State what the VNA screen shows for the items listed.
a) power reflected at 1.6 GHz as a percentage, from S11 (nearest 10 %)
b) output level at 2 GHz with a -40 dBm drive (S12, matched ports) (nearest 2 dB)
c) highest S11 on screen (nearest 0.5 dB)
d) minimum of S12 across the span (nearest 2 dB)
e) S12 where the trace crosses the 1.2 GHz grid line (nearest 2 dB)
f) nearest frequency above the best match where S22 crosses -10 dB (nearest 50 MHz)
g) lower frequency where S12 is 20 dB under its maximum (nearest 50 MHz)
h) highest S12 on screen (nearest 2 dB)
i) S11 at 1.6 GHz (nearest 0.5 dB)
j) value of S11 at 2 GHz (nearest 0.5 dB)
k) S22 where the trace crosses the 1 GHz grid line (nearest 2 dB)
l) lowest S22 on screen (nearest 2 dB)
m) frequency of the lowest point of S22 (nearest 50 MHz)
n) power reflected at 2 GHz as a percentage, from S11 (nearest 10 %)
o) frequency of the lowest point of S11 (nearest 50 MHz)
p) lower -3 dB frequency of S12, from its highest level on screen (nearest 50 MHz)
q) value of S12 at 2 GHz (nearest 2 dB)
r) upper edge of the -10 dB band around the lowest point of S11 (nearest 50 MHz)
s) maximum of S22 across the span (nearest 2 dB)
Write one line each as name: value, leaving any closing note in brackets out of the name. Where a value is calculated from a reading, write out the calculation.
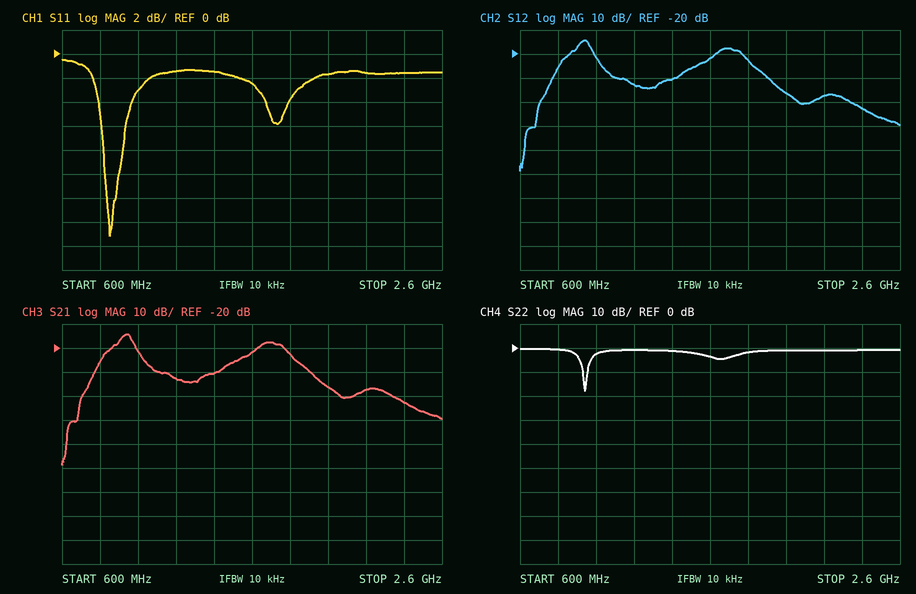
power reflected at 1.6 GHz as a percentage, from S11: 10^(-2.5/10) ≈ 56.2 %, so 60 % to the nearest 10 %
output level at 2 GHz with a -40 dBm drive (S12, matched ports): -40 dBm + (-36 dB) = -76 dBm
highest S11 on screen: -0.5 dB
minimum of S12 across the span: -68 dB
S12 where the trace crosses the 1.2 GHz grid line: -32 dB
nearest frequency above the best match where S22 crosses -10 dB: 950 MHz
lower frequency where S12 is 20 dB under its maximum: 750 MHz
highest S12 on screen: -14 dB
S11 at 1.6 GHz: -2.5 dB
value of S11 at 2 GHz: -1.5 dB
S22 where the trace crosses the 1 GHz grid line: -2 dB
lowest S22 on screen: -18 dB
frequency of the lowest point of S22: 950 MHz
power reflected at 2 GHz as a percentage, from S11: 10^(-1.5/10) ≈ 70.8 %, so 70 % to the nearest 10 %
frequency of the lowest point of S11: 850 MHz
lower -3 dB frequency of S12, from its highest level on screen: 900 MHz
value of S12 at 2 GHz: -36 dB
upper edge of the -10 dB band around the lowest point of S11: 900 MHz
maximum of S22 across the span: 0 dB
